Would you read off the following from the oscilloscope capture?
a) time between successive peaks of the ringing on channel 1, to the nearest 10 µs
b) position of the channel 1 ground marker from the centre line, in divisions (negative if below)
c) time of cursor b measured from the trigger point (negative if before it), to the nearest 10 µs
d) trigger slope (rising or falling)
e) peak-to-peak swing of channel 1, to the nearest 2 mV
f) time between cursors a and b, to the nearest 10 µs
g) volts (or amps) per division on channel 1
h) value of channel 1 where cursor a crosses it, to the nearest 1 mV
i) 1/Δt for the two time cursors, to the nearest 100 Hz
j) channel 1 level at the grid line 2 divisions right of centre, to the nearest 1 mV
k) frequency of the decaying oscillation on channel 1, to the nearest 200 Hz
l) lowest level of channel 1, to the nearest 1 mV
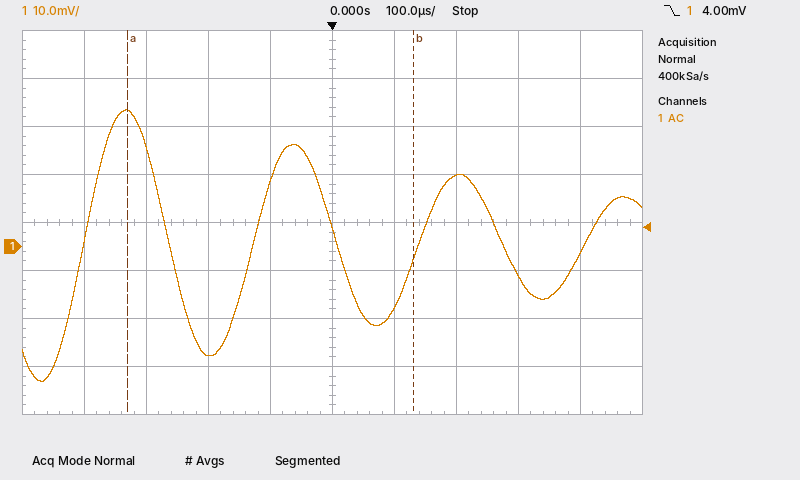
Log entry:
270 µs
-0.5 div
+130 µs
falling
56 mV
460 µs
10 mV
28 mV
2.2 kHz
15 mV
3.8 kHz
-28 mV
